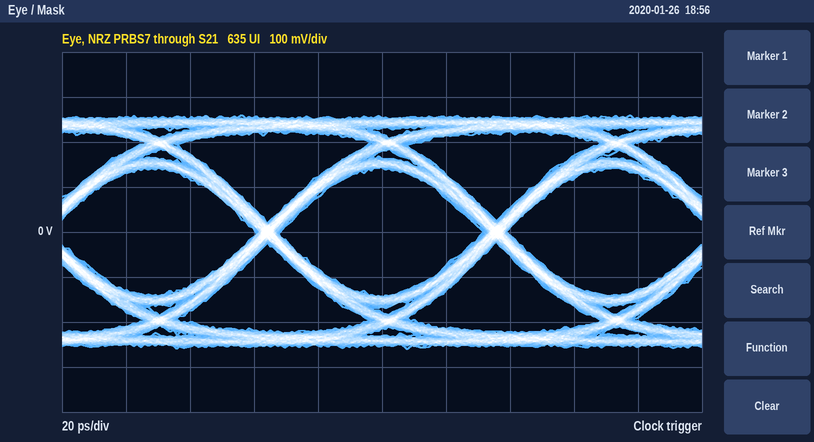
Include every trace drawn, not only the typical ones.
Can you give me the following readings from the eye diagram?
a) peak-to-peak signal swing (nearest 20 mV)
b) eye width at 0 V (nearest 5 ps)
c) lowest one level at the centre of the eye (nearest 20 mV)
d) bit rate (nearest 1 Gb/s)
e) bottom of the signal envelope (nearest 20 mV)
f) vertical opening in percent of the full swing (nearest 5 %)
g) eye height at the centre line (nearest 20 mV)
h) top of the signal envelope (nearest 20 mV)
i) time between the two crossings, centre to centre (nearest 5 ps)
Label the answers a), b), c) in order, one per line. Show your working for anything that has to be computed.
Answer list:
a) 520 mV
b) 65 ps
c) 140 mV
d) 14 Gb/s
e) -260 mV
f) 280 mV / 520 mV ≈ 53.8 %, so 55 % to the nearest 5 %
g) 280 mV
h) 260 mV
i) 70 ps
